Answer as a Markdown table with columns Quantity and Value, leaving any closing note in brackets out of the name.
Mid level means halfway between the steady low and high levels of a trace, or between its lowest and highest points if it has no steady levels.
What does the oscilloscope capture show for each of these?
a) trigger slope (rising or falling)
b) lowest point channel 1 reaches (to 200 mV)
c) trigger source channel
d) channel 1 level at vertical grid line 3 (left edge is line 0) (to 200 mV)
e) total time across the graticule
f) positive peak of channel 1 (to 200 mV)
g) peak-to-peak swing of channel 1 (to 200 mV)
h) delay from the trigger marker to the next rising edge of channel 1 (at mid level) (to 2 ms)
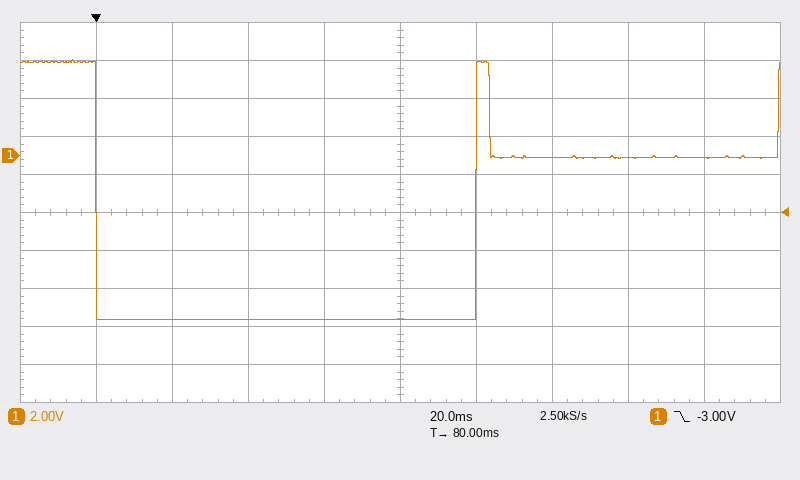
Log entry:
| Quantity | Value |
|---|---|
| trigger slope | falling |
| lowest point channel 1 reaches | -8.6 V |
| trigger source channel | channel 1 |
| channel 1 level at vertical grid line 3 (left edge is line 0) | -8.6 V |
| total time across the graticule | 200 ms |
| positive peak of channel 1 | 5.0 V |
| peak-to-peak swing of channel 1 | 13.6 V |
| delay from the trigger marker to the next rising edge of channel 1 (at mid level) | 100 ms |
